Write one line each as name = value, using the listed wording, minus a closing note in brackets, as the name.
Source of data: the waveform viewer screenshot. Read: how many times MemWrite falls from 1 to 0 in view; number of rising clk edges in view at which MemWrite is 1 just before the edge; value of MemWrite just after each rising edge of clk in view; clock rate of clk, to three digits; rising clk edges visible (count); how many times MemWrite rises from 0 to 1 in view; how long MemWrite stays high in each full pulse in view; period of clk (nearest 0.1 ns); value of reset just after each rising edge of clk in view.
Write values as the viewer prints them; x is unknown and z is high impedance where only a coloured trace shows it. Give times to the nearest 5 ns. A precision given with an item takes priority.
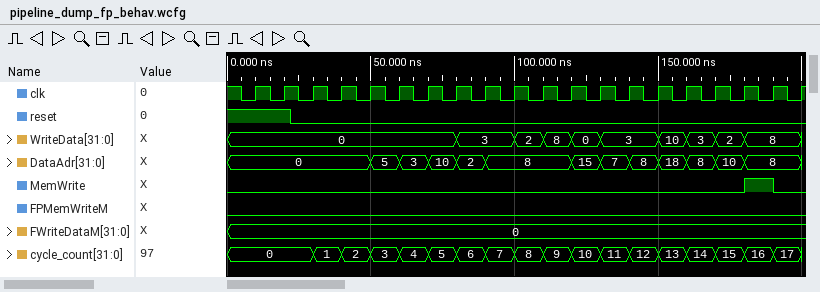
how many times MemWrite falls from 1 to 0 in view = 1
number of rising clk edges in view at which MemWrite is 1 just before the edge = 1
value of MemWrite just after each rising edge of clk in view = 0 0 0 0 0 0 0 0 0 0 0 0 0 0 0 0 0 1 0 0
clock rate of clk, to three digits = 100 MHz
rising clk edges visible = 20
how many times MemWrite rises from 0 to 1 in view = 1
how long MemWrite stays high in each full pulse in view = 10 ns
period of clk = 10 ns
value of reset just after each rising edge of clk in view = 1 1 0 0 0 0 0 0 0 0 0 0 0 0 0 0 0 0 0 0
